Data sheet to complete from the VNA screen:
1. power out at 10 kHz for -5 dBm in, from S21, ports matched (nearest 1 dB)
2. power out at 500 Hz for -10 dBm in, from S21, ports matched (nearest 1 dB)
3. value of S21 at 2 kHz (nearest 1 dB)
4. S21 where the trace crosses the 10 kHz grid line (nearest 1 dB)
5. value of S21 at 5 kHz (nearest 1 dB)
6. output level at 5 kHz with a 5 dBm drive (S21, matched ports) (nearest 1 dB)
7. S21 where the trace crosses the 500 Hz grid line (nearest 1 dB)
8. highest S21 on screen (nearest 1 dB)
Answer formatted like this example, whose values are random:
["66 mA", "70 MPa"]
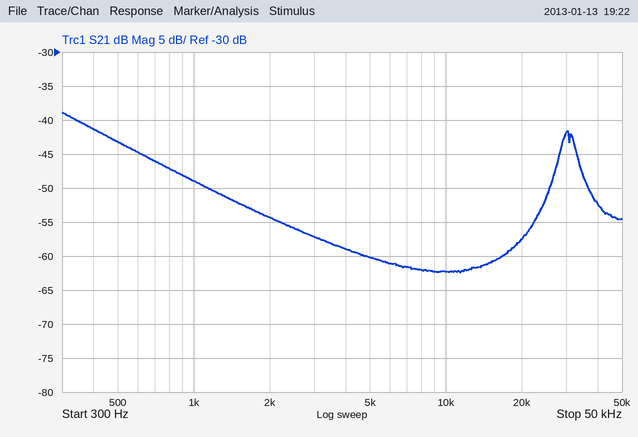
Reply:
["-67 dBm", "-53 dBm", "-54 dB", "-62 dB", "-60 dB", "-55 dBm", "-43 dB", "-39 dB"]
